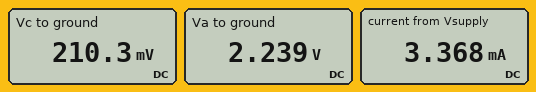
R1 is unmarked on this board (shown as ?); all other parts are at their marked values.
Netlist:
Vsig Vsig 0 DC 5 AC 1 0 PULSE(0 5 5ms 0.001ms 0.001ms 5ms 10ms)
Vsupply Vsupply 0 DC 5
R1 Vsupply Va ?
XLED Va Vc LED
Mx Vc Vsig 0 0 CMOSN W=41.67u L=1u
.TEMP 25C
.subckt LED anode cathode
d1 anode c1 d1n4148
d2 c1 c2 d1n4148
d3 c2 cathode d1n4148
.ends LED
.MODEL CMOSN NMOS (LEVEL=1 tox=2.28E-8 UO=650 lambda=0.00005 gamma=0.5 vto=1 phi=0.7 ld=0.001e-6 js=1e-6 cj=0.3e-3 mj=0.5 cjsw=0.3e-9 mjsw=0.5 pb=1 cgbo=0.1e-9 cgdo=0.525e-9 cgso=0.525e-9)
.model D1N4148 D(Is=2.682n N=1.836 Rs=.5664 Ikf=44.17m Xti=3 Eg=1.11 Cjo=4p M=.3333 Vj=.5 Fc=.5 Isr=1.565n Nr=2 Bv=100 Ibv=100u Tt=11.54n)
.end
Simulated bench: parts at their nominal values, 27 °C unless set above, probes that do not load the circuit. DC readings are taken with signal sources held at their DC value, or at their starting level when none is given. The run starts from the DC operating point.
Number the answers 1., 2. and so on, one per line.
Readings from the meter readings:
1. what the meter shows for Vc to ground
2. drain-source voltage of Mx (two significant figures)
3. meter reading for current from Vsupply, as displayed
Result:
1. 210.3 mV
2. 210 mV
3. 3.368 mA
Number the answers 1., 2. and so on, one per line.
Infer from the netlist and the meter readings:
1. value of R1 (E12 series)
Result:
1. 820 Ω
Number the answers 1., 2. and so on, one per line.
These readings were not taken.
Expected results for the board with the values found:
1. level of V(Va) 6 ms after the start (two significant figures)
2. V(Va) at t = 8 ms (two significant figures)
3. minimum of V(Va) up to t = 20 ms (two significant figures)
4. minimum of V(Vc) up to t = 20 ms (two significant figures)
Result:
1. 2.2 V
2. 2.2 V
3. 2.2 V
4. 210 mV
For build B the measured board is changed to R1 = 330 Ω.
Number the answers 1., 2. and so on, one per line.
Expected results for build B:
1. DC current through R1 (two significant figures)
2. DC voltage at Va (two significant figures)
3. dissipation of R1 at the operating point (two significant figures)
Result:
1. 7.2 mA
2. 2.6 V
3. 17 mW
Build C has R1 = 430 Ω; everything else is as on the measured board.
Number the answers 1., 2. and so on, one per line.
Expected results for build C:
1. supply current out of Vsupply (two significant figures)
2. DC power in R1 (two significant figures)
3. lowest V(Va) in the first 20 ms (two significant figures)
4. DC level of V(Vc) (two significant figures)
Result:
1. 5.8 mA
2. 15 mW
3. 2.5 V
4. 370 mV
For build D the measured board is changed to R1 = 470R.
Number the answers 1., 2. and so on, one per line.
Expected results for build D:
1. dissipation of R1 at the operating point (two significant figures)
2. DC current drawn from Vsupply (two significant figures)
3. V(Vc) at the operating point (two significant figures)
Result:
1. 14 mW
2. 5.4 mA
3. 340 mV
